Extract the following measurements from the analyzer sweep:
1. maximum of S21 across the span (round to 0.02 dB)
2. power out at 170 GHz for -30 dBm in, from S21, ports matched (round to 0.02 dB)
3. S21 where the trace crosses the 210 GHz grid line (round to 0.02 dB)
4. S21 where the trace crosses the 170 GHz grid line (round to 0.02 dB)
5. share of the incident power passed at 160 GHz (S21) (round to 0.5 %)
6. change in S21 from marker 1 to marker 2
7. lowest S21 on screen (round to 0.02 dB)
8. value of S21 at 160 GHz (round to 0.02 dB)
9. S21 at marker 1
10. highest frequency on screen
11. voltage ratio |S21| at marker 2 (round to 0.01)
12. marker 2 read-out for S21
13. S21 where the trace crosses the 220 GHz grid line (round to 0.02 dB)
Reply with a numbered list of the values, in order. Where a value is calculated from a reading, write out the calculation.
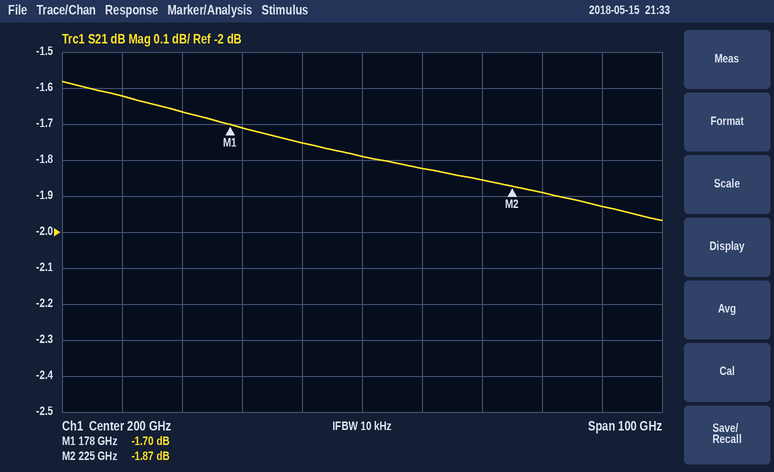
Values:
1. -1.58 dB
2. -30 dBm + (-1.66 dB) = -31.66 dBm
3. -1.82 dB
4. -1.66 dB
5. 10^(-1.62/10) ≈ 68.9 %, so 69.0 % to the nearest 0.5 %
6. -1.87 − (-1.7) = -0.17 dB
7. -1.96 dB
8. -1.62 dB
9. -1.70 dB
10. 250 GHz
11. 10^(-1.87/20) ≈ 0.81
12. -1.87 dB
13. -1.86 dB
